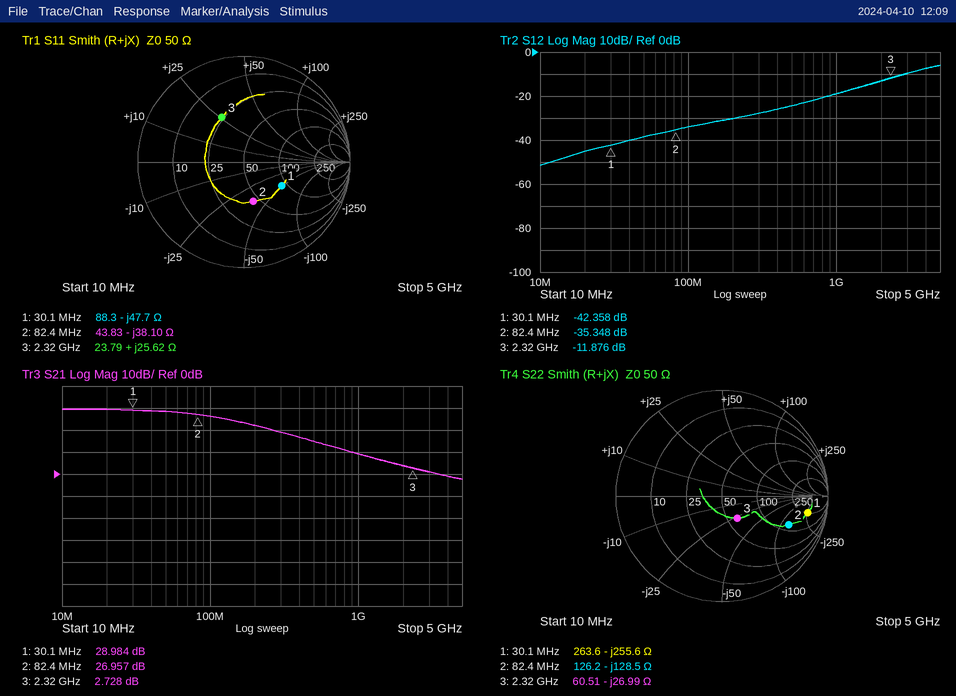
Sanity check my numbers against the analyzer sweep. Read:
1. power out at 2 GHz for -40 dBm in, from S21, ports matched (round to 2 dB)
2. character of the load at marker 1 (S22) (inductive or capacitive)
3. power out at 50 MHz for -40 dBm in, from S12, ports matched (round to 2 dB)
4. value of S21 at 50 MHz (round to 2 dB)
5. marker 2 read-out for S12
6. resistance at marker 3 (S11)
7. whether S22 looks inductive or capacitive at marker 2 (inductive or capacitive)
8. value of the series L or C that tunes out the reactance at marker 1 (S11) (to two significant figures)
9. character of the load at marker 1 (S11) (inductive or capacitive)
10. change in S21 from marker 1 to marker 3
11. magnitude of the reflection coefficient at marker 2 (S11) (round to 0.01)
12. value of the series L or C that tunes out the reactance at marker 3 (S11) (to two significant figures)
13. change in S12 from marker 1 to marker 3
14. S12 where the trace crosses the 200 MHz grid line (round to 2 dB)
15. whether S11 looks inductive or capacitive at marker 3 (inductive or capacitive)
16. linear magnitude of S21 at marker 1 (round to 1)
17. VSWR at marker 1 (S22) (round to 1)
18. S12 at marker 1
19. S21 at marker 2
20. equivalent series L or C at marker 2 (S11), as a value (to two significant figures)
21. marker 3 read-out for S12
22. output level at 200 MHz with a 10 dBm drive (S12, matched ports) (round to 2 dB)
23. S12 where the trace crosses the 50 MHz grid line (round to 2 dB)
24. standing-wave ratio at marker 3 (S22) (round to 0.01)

-36 dBm
capacitive
-78 dBm
28 dB
-35.348 dB
23.79 Ω
capacitive
250 nH
capacitive
-26.256 dB
0.38
2.7 pF
30.482 dB
-30 dB
inductive
28
10
-42.358 dB
26.957 dB
51 pF
-11.876 dB
-20 dBm
-38 dB
1.68
